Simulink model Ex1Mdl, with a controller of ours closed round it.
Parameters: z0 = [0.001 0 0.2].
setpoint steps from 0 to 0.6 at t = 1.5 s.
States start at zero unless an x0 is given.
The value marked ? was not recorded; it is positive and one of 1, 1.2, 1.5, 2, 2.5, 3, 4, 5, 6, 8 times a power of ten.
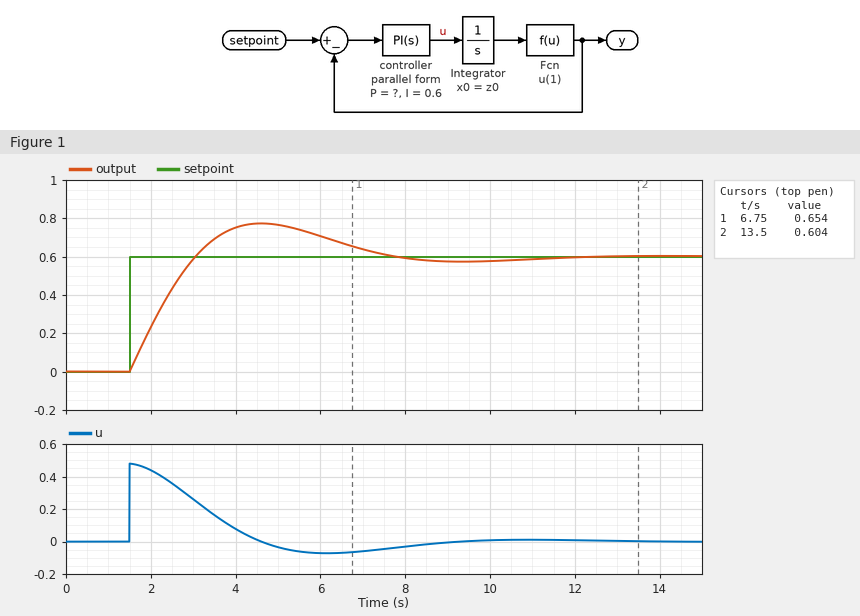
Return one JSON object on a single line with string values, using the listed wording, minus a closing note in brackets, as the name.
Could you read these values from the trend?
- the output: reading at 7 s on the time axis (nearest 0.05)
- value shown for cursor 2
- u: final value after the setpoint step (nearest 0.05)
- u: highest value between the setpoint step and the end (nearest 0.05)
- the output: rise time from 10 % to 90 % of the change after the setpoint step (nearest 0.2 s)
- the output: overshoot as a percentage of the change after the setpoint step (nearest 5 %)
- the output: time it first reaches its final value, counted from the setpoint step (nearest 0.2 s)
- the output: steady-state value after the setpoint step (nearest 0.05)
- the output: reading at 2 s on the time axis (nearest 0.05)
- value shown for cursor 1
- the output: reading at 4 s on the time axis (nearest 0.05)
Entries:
{"the output: reading at 7 s on the time axis": "0.65", "value shown for cursor 2": "0.604", "u: final value after the setpoint step": "0.00", "u: highest value between the setpoint step and the end": "0.50", "the output: rise time from 10 % to 90 % of the change after the setpoint step": "1.2 s", "the output: overshoot as a percentage of the change after the setpoint step": "30 %", "the output: time it first reaches its final value, counted from the setpoint step": "1.6 s", "the output: steady-state value after the setpoint step": "0.60", "the output: reading at 2 s on the time axis": "0.25", "value shown for cursor 1": "0.654", "the output: reading at 4 s on the time axis": "0.75"}
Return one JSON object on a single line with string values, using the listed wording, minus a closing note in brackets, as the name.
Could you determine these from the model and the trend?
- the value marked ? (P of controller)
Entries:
{"the value marked ?": "0.8"}
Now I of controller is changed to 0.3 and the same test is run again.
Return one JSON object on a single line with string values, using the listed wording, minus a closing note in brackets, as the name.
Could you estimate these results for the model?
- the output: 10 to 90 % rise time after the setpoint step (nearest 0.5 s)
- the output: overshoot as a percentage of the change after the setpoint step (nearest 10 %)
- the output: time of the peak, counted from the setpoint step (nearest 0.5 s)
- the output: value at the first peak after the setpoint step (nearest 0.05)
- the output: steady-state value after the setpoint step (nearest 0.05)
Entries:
{"the output: 10 to 90 % rise time after the setpoint step": "1.5 s", "the output: overshoot as a percentage of the change after the setpoint step": "20 %", "the output: time of the peak, counted from the setpoint step": "4.0 s", "the output: value at the first peak after the setpoint step": "0.70", "the output: steady-state value after the setpoint step": "0.60"}
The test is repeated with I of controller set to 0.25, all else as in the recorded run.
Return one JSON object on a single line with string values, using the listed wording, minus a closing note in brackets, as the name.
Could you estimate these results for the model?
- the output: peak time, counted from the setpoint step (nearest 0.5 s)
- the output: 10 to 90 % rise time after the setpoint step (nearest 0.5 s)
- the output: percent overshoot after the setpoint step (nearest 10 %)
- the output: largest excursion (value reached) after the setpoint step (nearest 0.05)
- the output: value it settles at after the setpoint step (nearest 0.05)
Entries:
{"the output: peak time, counted from the setpoint step": "4.5 s", "the output: 10 to 90 % rise time after the setpoint step": "1.5 s", "the output: percent overshoot after the setpoint step": "20 %", "the output: largest excursion (value reached) after the setpoint step": "0.70", "the output: value it settles at after the setpoint step": "0.60"}
